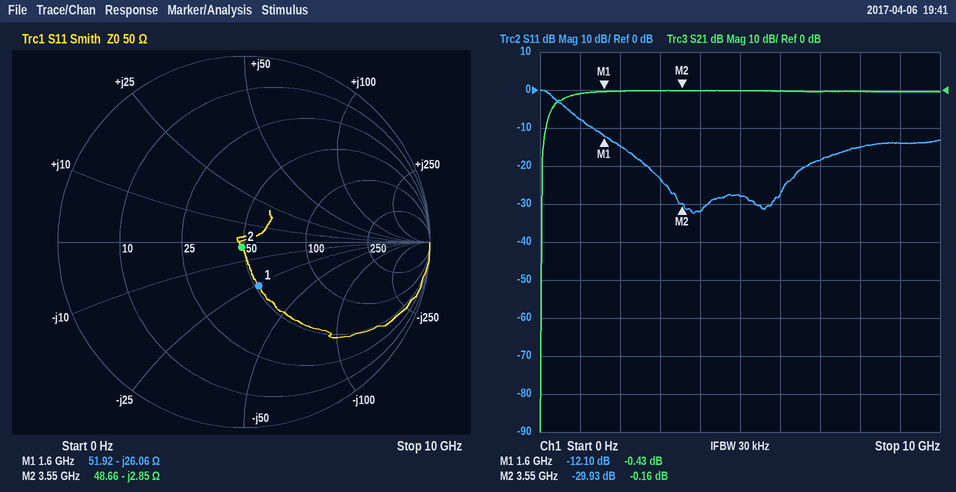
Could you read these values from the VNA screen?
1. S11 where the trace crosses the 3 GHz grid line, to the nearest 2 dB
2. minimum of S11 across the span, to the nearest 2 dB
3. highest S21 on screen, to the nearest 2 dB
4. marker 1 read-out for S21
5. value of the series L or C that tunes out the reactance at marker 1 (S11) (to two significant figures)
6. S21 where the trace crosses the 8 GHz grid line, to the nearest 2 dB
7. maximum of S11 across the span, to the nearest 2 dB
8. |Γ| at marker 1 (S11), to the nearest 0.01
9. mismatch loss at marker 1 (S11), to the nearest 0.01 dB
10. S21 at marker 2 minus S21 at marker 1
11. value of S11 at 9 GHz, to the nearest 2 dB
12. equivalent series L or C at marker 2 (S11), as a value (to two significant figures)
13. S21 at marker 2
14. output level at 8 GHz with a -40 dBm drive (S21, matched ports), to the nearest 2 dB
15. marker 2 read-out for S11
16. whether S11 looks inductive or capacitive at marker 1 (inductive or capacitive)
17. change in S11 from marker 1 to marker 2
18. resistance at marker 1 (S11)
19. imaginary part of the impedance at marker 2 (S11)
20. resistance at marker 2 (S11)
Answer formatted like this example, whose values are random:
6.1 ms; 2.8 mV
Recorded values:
-24 dB; -32 dB; 0 dB; -0.43 dB; 2.6 nH; 0 dB; 0 dB; 0.25; 0.28 dB; 0.27 dB; -14 dB; 16 pF; -0.16 dB; -40 dBm; -29.93 dB; capacitive; -17.83 dB; 51.92 Ω; -2.85 Ω; 48.66 Ω
